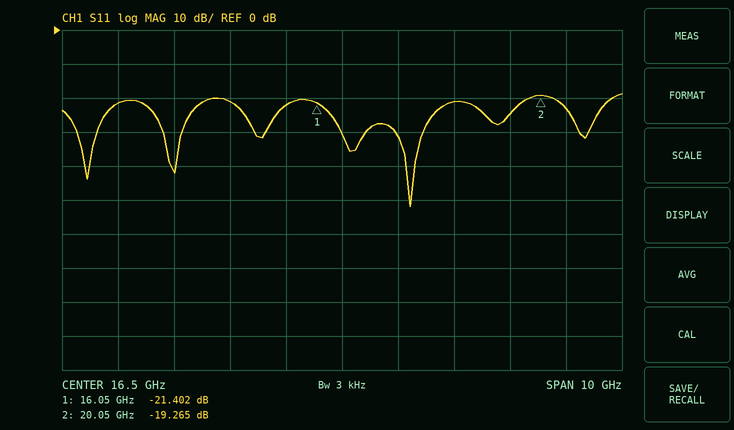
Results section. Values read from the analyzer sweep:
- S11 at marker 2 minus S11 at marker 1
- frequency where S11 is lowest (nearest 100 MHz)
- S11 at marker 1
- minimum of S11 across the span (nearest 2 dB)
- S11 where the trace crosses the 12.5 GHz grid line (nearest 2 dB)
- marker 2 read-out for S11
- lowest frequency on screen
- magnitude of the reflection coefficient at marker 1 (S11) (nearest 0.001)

2.137 dB
17.7 GHz
-21.402 dB
-52 dB
-22 dB
-19.265 dB
11.5 GHz
0.085
